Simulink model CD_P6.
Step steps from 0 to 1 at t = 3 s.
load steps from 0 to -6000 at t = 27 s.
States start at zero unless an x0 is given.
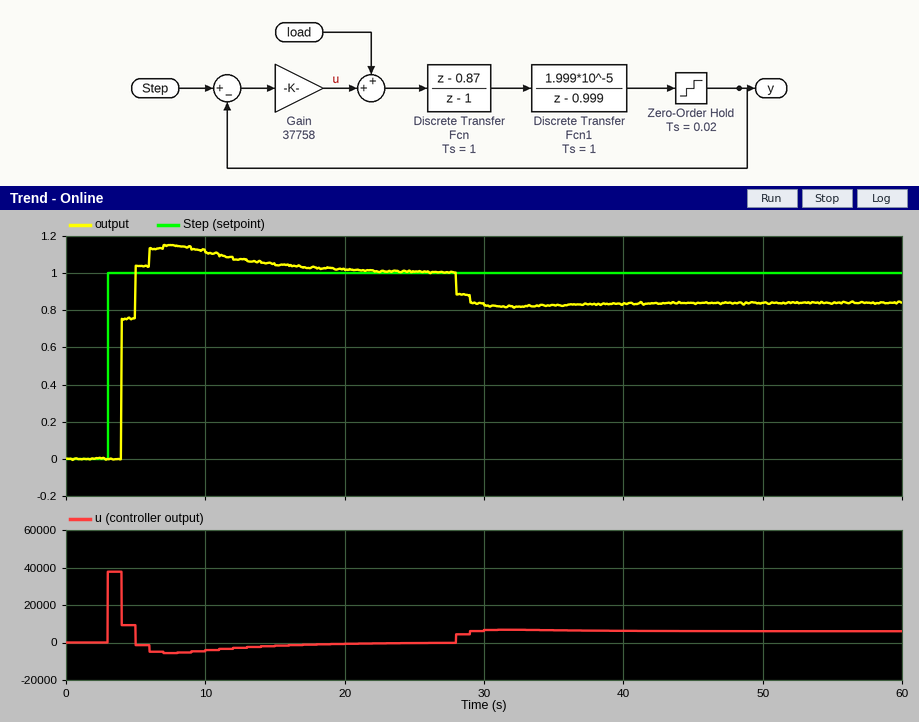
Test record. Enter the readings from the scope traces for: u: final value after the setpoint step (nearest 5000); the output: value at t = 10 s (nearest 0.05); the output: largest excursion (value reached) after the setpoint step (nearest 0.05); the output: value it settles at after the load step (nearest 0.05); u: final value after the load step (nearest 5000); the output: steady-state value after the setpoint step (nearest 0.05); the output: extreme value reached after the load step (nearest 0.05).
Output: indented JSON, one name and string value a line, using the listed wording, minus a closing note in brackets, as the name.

{
  "u: final value after the setpoint step": "0",
  "the output: value at t = 10 s": "1.10",
  "the output: largest excursion (value reached) after the setpoint step": "1.15",
  "the output: value it settles at after the load step": "0.85",
  "u: final value after the load step": "5000",
  "the output: steady-state value after the setpoint step": "1.00",
  "the output: extreme value reached after the load step": "0.80"
}
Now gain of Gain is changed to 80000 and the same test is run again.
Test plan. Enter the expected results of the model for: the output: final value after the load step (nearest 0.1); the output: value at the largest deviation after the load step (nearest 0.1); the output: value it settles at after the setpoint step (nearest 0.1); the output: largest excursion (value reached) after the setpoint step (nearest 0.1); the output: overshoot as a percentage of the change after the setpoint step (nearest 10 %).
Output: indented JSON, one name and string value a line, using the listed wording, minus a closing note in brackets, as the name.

{
  "the output: final value after the load step": "0.9",
  "the output: value at the largest deviation after the load step": "0.9",
  "the output: value it settles at after the setpoint step": "1.0",
  "the output: largest excursion (value reached) after the setpoint step": "1.6",
  "the output: overshoot as a percentage of the change after the setpoint step": "60 %"
}
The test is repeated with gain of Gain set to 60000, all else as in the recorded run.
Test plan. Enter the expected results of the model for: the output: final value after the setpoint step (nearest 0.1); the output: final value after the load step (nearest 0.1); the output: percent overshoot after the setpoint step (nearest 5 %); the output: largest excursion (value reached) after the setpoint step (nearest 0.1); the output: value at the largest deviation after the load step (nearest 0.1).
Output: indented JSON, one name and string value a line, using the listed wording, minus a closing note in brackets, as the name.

{
  "the output: final value after the setpoint step": "1.0",
  "the output: final value after the load step": "0.9",
  "the output: percent overshoot after the setpoint step": "20 %",
  "the output: largest excursion (value reached) after the setpoint step": "1.2",
  "the output: value at the largest deviation after the load step": "0.9"
}
